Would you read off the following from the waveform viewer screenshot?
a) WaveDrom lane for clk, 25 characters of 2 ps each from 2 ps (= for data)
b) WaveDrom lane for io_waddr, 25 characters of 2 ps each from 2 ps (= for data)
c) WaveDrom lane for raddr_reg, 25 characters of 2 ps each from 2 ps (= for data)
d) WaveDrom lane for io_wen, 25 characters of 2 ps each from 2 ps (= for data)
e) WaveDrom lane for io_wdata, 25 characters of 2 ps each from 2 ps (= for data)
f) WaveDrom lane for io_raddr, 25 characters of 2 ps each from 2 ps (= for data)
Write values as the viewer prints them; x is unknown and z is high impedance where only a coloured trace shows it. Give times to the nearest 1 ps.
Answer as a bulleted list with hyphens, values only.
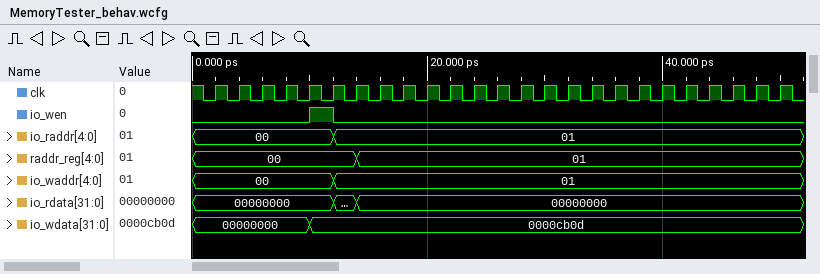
- {name: 'clk', wave: 'p........................'}
- {name: 'io_waddr', wave: '=....=...................', data: '00 01'}
- {name: 'raddr_reg', wave: '=.....=..................', data: '00 01'}
- {name: 'io_wen', wave: '0...10...................'}
- {name: 'io_wdata', wave: '=...=....................', data: '00000000 0000cb0d'}
- {name: 'io_raddr', wave: '=....=...................', data: '00 01'}
